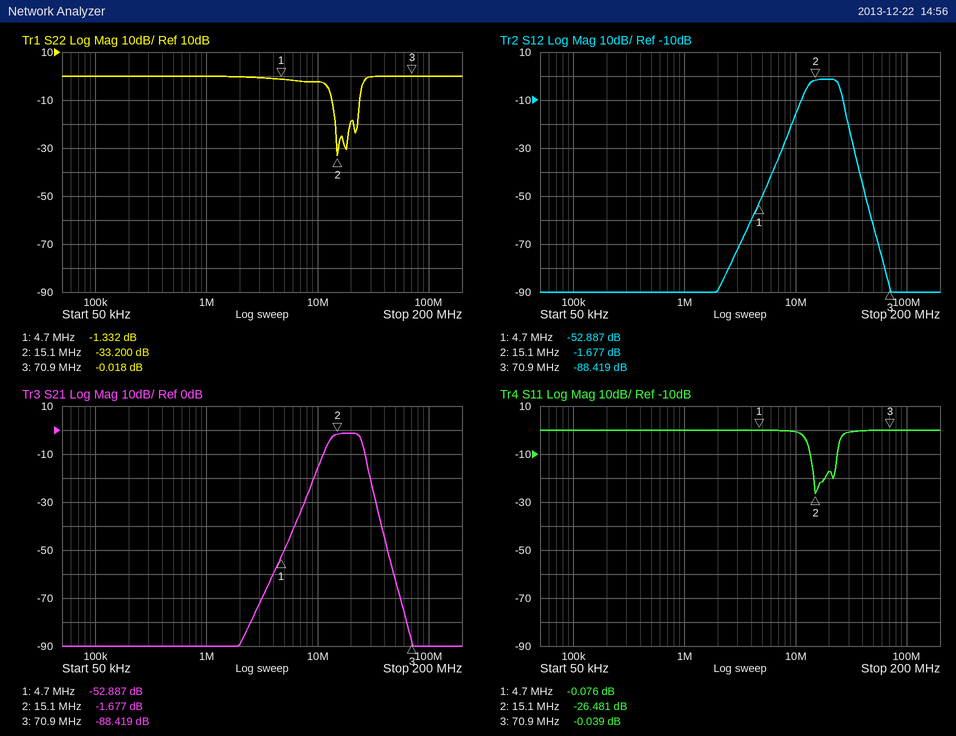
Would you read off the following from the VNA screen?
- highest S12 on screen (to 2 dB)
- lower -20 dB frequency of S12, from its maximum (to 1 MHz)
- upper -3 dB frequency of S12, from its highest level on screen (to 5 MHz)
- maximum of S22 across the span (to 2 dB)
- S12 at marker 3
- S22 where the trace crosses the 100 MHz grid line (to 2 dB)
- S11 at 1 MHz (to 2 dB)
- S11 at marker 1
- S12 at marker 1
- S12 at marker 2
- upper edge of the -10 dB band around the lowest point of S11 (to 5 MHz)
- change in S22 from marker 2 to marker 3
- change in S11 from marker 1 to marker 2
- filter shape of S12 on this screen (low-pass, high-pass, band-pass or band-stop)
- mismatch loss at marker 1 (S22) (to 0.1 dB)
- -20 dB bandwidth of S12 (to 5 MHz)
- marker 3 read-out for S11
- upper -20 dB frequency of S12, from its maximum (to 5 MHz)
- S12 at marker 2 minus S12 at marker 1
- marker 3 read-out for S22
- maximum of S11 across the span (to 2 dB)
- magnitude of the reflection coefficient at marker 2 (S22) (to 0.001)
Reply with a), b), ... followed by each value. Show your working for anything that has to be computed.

a) -2 dB
b) 9 MHz
c) 25 MHz
d) 0 dB
e) -88.419 dB
f) 0 dB
g) 0 dB
h) -0.076 dB
i) -52.887 dB
j) -1.677 dB
k) 25 MHz
l) -0.018 − (-33.2) = 33.182 dB
m) -26.481 − (-0.076) = -26.405 dB
n) band-pass
o) −10 log10(1 − 10^(-1.332/10)) ≈ 5.8 dB
p) 30 MHz − 9 MHz = 21 MHz
q) -0.039 dB
r) 30 MHz
s) -1.677 − (-52.887) = 51.210 dB
t) -0.018 dB
u) 0 dB
v) 10^(-33.2/20) ≈ 0.022
